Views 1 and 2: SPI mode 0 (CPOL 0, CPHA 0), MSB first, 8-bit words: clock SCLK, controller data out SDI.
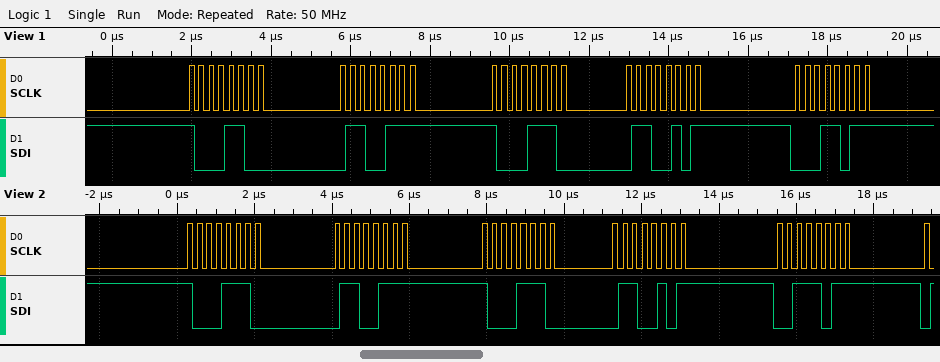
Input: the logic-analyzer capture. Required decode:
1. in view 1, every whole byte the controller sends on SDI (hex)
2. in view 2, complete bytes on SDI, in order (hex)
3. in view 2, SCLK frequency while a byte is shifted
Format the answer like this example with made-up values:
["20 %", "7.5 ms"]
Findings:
["8C 67 8E 65 1B", "8E 67 8E 65 3B", "4 MHz"]
